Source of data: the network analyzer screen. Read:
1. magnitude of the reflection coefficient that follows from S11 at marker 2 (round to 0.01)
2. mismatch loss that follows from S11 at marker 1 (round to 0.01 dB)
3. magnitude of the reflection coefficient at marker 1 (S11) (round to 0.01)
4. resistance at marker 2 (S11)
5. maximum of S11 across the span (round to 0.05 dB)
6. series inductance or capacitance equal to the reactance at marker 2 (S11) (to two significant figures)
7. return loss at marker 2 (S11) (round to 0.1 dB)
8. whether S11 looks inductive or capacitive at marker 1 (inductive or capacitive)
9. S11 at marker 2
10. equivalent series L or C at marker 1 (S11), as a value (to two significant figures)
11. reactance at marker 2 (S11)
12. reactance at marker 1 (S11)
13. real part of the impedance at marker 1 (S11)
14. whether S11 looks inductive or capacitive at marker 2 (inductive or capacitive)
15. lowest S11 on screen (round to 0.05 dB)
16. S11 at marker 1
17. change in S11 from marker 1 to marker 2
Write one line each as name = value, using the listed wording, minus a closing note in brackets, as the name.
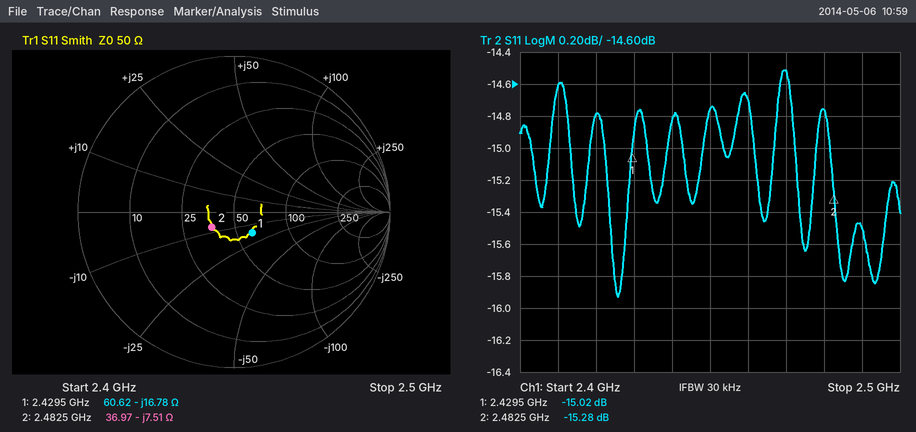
magnitude of the reflection coefficient that follows from S11 at marker 2 = 0.17
mismatch loss that follows from S11 at marker 1 = 0.14 dB
magnitude of the reflection coefficient at marker 1 (S11) = 0.18
resistance at marker 2 = 36.97 Ω
maximum of S11 across the span = -14.50 dB
series inductance or capacitance equal to the reactance at marker 2 (S11) = 8.5 pF
return loss at marker 2 (S11) = 15.3 dB
whether S11 looks inductive or capacitive at marker 1 = capacitive
S11 at marker 2 = -15.28 dB
equivalent series L or C at marker 1 (S11), as a value = 3.9 pF
reactance at marker 2 = -7.51 Ω
reactance at marker 1 = -16.78 Ω
real part of the impedance at marker 1 = 60.62 Ω
whether S11 looks inductive or capacitive at marker 2 = capacitive
lowest S11 on screen = -15.95 dB
S11 at marker 1 = -15.02 dB
change in S11 from marker 1 to marker 2 = -0.26 dB
